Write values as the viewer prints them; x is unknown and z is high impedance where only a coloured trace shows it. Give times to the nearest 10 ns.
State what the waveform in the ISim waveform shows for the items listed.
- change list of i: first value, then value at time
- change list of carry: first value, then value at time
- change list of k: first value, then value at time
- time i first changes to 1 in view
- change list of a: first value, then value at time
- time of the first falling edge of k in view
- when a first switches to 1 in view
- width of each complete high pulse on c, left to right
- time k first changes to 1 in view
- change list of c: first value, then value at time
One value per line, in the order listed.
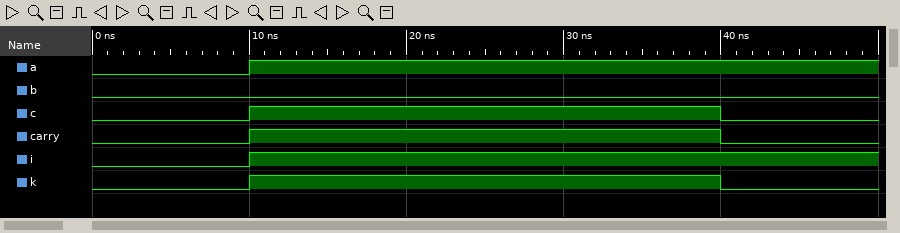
0, 1 at 10 ns
0, 1 at 10 ns, 0 at 40 ns
0, 1 at 10 ns, 0 at 40 ns
10 ns
0, 1 at 10 ns
40 ns
10 ns
30 ns
10 ns
0, 1 at 10 ns, 0 at 40 ns
